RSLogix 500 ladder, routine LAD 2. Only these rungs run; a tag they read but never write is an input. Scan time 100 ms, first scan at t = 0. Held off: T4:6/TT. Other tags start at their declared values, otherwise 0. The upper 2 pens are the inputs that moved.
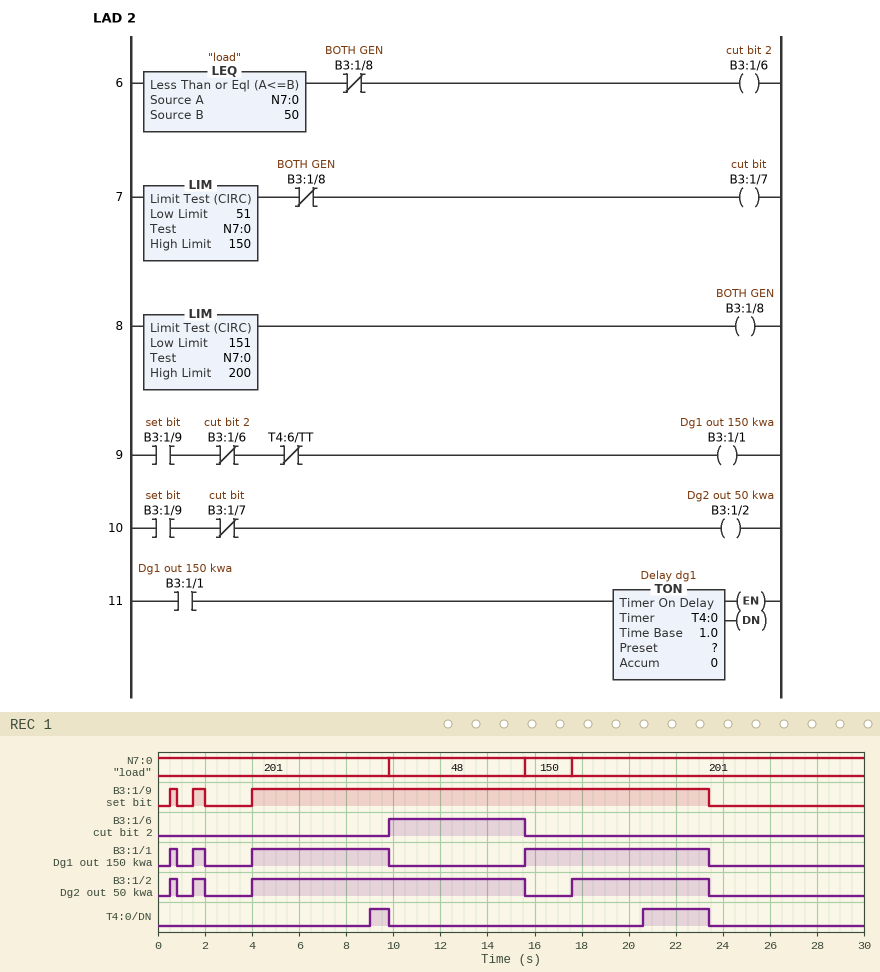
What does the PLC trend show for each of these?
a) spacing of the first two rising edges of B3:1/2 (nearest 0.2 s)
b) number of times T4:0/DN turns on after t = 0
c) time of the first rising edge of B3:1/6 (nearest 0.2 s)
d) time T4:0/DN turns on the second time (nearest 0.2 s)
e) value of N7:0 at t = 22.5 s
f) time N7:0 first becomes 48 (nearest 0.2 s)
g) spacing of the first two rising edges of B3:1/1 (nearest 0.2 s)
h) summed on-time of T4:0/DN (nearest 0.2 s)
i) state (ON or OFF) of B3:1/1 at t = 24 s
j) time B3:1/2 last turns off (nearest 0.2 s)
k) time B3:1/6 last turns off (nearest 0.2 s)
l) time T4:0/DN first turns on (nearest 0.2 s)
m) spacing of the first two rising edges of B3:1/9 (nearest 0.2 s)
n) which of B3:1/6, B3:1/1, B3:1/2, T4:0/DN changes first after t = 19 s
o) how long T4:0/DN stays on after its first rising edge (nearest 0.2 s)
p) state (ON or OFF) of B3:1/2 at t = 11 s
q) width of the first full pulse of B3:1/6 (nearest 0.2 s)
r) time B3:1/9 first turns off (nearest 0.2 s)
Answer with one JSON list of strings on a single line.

["1.0 s", "2", "9.8 s", "20.6 s", "201", "9.8 s", "1.0 s", "3.6 s", "OFF", "23.4 s", "15.6 s", "9.0 s", "1.0 s", "T4:0/DN", "0.8 s", "ON", "5.8 s", "0.8 s"]
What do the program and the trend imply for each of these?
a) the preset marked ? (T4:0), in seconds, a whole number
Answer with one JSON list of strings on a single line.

["5 s"]
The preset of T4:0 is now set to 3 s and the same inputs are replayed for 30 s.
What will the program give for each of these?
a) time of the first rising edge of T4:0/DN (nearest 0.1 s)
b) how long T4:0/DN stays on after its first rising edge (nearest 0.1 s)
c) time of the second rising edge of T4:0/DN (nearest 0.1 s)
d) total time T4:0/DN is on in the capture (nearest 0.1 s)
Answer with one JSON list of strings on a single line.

["7.0 s", "2.8 s", "18.6 s", "7.6 s"]
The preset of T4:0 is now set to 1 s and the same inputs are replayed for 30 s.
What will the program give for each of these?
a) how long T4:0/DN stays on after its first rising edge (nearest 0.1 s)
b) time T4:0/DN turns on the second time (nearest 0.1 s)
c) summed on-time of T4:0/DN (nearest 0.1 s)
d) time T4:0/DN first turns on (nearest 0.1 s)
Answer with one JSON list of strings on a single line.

["4.8 s", "16.6 s", "11.6 s", "5.0 s"]
